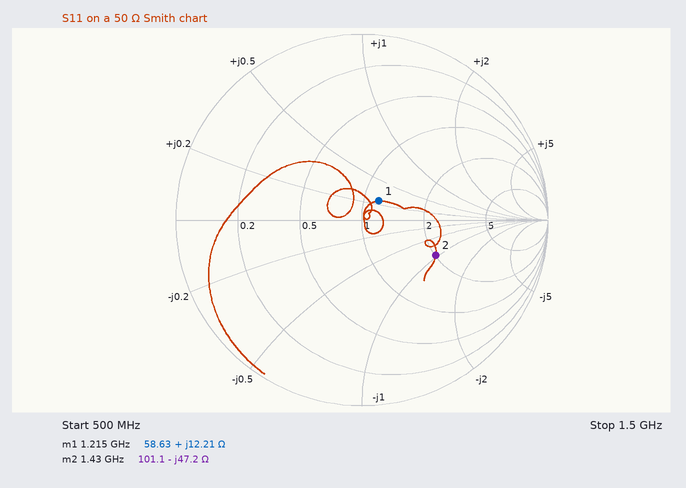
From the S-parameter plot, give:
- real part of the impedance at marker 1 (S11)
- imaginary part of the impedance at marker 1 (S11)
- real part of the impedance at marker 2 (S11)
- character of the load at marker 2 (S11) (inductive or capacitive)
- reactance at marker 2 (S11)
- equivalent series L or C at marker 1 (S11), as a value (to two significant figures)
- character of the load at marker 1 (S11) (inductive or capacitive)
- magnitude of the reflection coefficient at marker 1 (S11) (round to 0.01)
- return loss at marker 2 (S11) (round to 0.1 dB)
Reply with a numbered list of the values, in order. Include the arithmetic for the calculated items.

1. 58.63 Ω
2. +12.21 Ω
3. 101.1 Ω
4. capacitive
5. -47.2 Ω
6. L = 12.21 Ω/(2π × 1.215 GHz) ≈ 1.6 nH
7. inductive
8. 0.14
9. 7.1 dB
